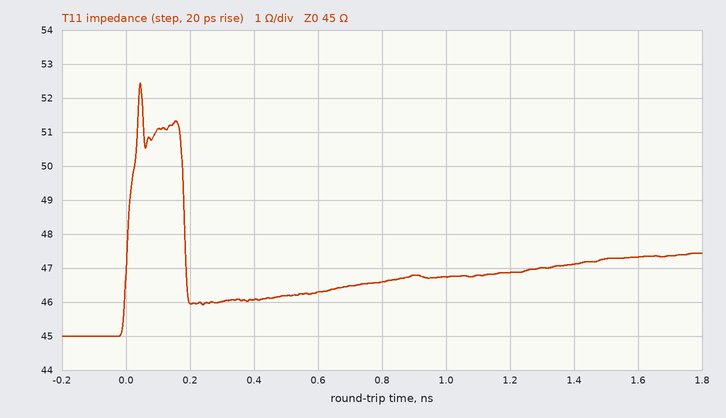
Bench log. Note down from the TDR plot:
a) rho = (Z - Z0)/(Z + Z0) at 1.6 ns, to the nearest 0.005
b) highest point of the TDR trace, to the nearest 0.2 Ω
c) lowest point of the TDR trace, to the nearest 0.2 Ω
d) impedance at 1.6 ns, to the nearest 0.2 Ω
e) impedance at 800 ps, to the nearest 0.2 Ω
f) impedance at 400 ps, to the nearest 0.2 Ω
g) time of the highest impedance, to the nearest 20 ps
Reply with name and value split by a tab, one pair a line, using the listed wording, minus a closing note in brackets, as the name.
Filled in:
rho = (Z - Z0)/(Z + Z0) at 1.6 ns, to the nearest 0.005	+0.025
highest point of the TDR trace, to the nearest 0.2 Ω	52.4 Ω
lowest point of the TDR trace, to the nearest 0.2 Ω	45.0 Ω
impedance at 1.6 ns, to the nearest 0.2 Ω	47.4 Ω
impedance at 800 ps, to the nearest 0.2 Ω	46.6 Ω
impedance at 400 ps, to the nearest 0.2 Ω	46.0 Ω
time of the highest impedance, to the nearest 20 ps	40 ps
